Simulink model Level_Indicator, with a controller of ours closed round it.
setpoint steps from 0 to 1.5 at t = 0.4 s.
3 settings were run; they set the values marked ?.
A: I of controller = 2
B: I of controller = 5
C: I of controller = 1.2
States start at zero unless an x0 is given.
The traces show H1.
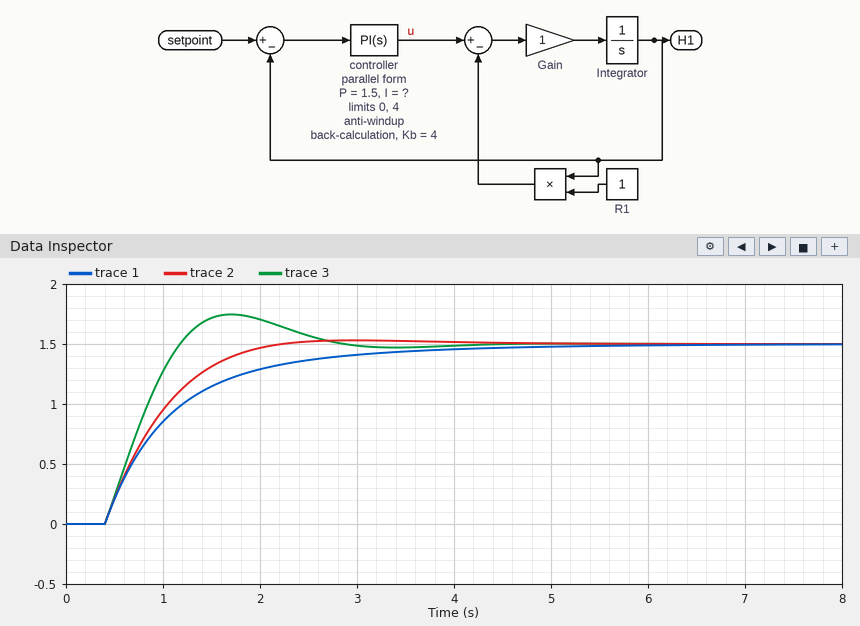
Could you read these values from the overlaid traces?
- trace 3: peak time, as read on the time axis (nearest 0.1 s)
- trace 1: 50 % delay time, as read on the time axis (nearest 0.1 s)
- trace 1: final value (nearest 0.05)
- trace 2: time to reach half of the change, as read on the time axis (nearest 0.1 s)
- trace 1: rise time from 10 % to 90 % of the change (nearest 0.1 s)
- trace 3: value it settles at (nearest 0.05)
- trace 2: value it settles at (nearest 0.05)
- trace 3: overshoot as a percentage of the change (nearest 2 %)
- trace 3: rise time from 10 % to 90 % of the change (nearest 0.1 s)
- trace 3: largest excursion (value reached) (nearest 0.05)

1.7 s
0.9 s
1.50
0.8 s
1.9 s
1.50
1.50
16 %
0.6 s
1.75
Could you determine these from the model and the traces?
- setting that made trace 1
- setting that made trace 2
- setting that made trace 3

C
A
B
